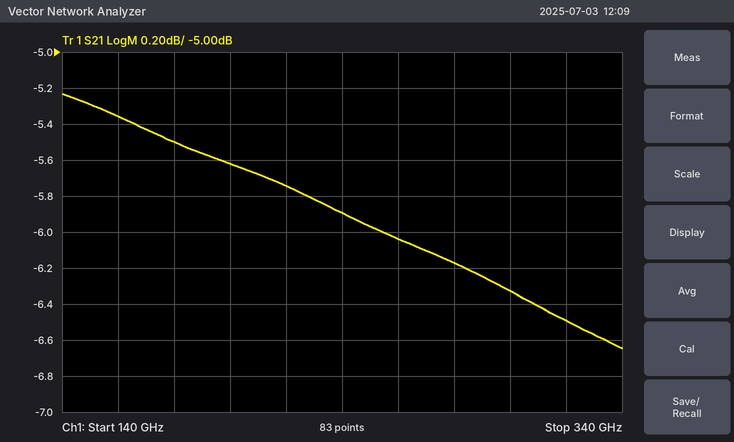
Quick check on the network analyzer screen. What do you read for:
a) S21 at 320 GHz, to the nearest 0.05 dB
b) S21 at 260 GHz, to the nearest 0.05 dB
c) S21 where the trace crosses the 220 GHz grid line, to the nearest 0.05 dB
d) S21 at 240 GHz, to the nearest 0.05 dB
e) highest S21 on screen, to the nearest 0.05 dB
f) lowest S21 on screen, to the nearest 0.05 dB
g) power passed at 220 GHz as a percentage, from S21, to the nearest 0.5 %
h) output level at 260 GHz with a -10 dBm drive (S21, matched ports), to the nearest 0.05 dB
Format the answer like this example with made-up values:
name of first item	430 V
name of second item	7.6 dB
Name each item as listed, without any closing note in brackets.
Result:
S21 at 320 GHz, to the nearest 0.05 dB	-6.50 dB
S21 at 260 GHz, to the nearest 0.05 dB	-6.05 dB
S21 where the trace crosses the 220 GHz grid line, to the nearest 0.05 dB	-5.75 dB
S21 at 240 GHz, to the nearest 0.05 dB	-5.90 dB
highest S21 on screen, to the nearest 0.05 dB	-5.25 dB
lowest S21 on screen, to the nearest 0.05 dB	-6.65 dB
power passed at 220 GHz as a percentage, from S21, to the nearest 0.5 %	26.5 %
output level at 260 GHz with a -10 dBm drive (S21, matched ports), to the nearest 0.05 dB	-16.05 dBm
